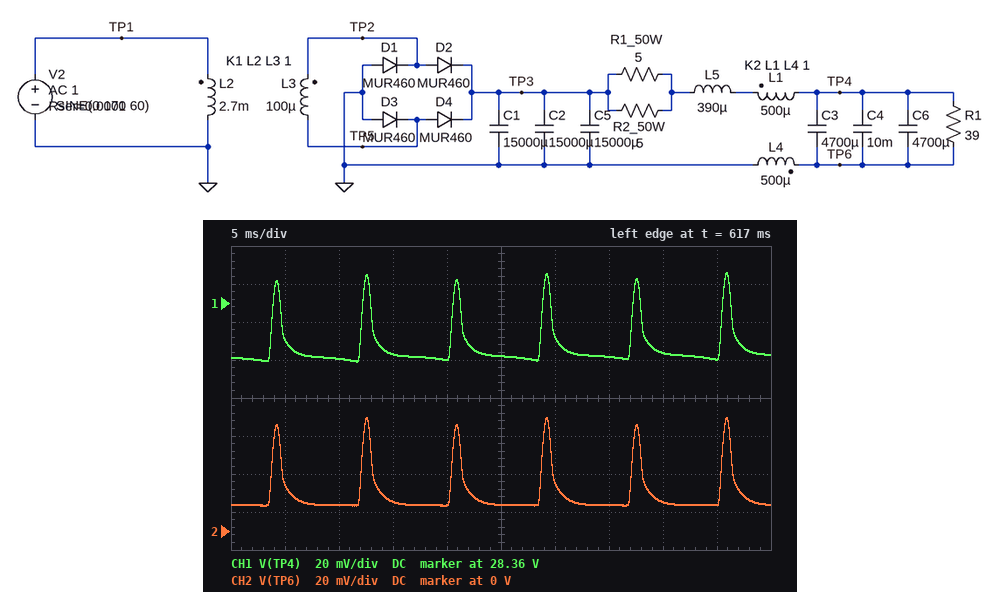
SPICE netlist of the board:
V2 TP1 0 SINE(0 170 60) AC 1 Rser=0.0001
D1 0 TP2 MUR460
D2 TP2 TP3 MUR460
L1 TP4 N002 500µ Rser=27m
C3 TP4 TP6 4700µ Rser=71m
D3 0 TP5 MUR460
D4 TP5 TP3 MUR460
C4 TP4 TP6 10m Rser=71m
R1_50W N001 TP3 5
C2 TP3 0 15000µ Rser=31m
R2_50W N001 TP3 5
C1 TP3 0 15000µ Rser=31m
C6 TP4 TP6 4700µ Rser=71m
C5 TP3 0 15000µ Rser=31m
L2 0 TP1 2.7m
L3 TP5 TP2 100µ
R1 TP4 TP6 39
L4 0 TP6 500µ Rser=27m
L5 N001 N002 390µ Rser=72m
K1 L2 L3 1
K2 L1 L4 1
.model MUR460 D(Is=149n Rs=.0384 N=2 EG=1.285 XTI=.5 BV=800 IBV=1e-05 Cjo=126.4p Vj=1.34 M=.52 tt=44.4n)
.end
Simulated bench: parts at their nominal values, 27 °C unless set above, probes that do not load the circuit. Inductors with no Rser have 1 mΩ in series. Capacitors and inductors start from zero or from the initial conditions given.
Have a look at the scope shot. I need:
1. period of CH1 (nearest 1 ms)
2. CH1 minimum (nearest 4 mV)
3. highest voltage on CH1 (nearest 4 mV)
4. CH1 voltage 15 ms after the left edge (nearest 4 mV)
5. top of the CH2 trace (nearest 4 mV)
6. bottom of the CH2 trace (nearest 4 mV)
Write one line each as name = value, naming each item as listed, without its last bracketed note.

period of CH1 = 8 ms
CH1 minimum = 28.328 V
highest voltage on CH1 = 28.376 V
CH1 voltage 15 ms after the left edge = 28.332 V
top of the CH2 trace = 60 mV
bottom of the CH2 trace = 12 mV
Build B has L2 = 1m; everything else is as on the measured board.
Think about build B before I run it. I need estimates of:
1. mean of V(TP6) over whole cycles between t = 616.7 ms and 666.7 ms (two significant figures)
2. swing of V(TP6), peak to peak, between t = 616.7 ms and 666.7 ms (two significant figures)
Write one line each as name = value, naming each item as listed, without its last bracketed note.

mean of V(TP6) over whole cycles between t = 616.7 ms and 666.7 ms = 33 mV
swing of V(TP6), peak to peak, between t = 616.7 ms and 666.7 ms = 81 mV
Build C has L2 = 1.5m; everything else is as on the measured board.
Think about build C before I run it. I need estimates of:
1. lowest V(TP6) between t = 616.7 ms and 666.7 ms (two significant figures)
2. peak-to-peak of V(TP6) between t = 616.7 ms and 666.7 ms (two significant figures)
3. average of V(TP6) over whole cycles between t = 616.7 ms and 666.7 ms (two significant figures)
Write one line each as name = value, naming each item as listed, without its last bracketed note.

lowest V(TP6) between t = 616.7 ms and 666.7 ms = 18 mV
peak-to-peak of V(TP6) between t = 616.7 ms and 666.7 ms = 65 mV
average of V(TP6) over whole cycles between t = 616.7 ms and 666.7 ms = 27 mV
